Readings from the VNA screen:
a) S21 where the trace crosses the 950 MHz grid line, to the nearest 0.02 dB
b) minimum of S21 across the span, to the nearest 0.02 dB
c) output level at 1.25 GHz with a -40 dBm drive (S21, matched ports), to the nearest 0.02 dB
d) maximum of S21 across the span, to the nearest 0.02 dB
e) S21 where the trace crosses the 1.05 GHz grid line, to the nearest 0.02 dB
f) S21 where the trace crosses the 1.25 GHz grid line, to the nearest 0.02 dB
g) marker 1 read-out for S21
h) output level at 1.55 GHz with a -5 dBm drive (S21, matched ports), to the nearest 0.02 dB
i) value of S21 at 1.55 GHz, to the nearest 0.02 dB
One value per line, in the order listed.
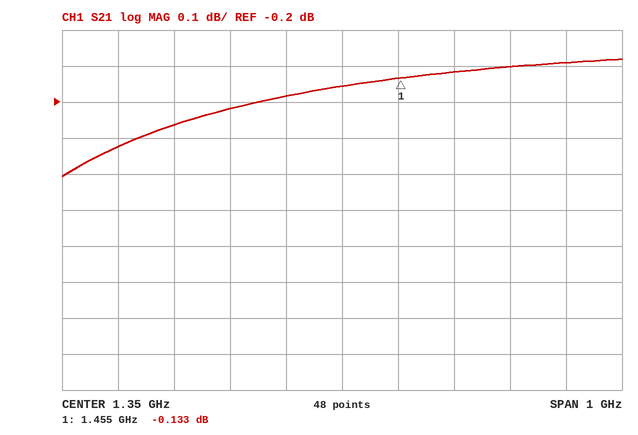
-0.32 dB
-0.40 dB
-40.18 dBm
-0.08 dB
-0.26 dB
-0.18 dB
-0.133 dB
-5.12 dBm
-0.12 dB
